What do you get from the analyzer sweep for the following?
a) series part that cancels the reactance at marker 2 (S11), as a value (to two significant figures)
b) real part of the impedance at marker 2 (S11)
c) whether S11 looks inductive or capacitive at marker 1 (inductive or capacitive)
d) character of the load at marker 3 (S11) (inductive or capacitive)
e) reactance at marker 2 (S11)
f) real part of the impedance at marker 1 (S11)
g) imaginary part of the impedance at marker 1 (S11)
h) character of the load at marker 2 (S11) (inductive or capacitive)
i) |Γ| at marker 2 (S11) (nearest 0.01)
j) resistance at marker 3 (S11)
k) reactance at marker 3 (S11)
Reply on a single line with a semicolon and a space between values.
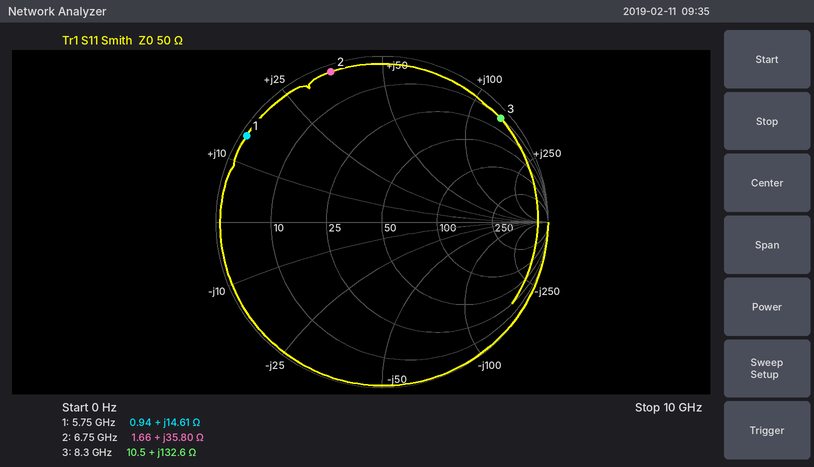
660 fF; 1.66 Ω; inductive; inductive; +35.80 Ω; 0.94 Ω; +14.61 Ω; inductive; 0.96; 10.5 Ω; +132.6 Ω
